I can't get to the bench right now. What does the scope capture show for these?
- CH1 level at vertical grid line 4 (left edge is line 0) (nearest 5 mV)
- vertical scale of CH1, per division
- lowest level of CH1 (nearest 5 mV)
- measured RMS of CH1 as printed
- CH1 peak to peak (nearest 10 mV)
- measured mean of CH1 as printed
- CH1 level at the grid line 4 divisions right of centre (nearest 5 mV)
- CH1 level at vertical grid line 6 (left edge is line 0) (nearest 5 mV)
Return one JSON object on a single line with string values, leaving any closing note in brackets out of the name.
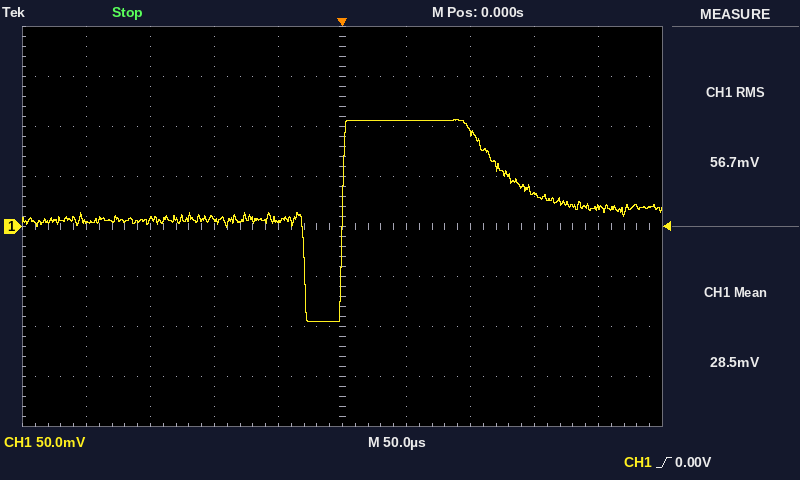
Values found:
{"CH1 level at vertical grid line 4 (left edge is line 0)": "5 mV", "vertical scale of CH1, per division": "50 mV", "lowest level of CH1": "-95 mV", "measured RMS of CH1 as printed": "56.7 mV", "CH1 peak to peak": "200 mV", "measured mean of CH1 as printed": "28.5 mV", "CH1 level at the grid line 4 divisions right of centre": "20 mV", "CH1 level at vertical grid line 6 (left edge is line 0)": "105 mV"}
